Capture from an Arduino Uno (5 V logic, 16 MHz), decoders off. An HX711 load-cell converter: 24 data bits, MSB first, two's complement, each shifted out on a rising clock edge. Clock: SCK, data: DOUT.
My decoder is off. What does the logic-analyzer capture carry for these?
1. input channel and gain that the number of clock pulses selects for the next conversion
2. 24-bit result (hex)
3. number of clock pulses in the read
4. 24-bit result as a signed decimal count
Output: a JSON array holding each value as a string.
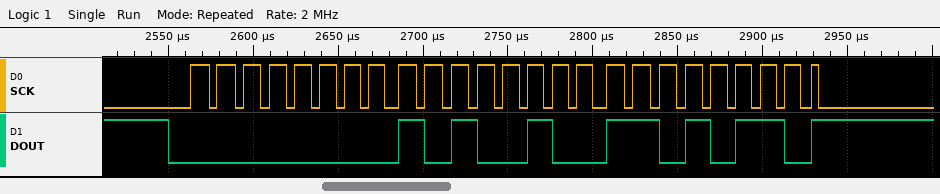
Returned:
["channel A, gain 128", "0x00A4D6", "25", "42198"]
